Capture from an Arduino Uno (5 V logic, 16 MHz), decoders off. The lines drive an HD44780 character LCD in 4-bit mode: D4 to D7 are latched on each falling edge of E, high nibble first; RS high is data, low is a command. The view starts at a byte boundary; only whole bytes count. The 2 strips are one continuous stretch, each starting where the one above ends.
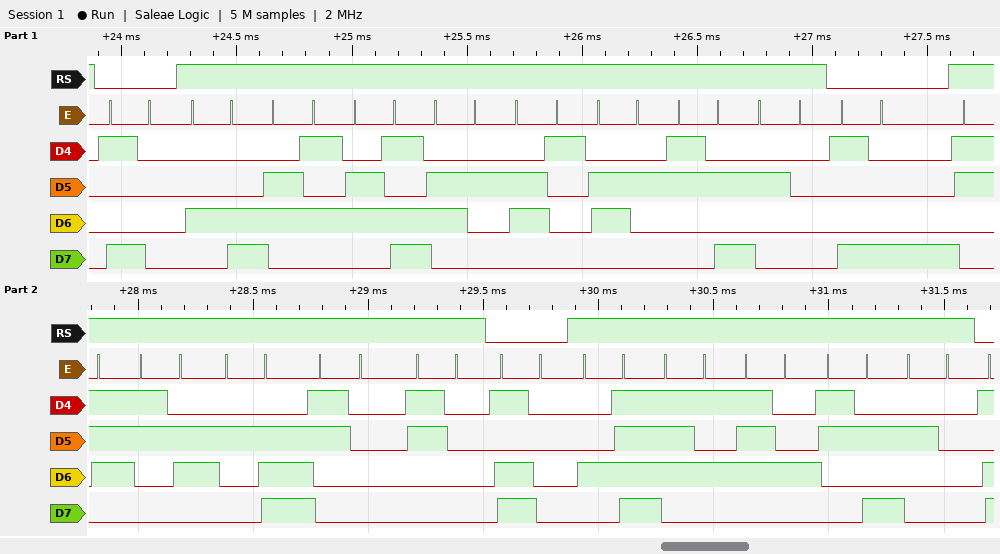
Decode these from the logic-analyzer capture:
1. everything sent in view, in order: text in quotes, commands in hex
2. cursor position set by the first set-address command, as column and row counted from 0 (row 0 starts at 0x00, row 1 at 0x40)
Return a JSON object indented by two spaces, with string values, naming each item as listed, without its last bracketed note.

{
  "everything sent in view, in order: text in quotes, commands in hex": "0x90 \"Lembab: \" 0x98 \"76.00\" 0xD0 \"Out: \"",
  "cursor position set by the first set-address command, as column and row counted from 0": "column 16, row 0"
}
